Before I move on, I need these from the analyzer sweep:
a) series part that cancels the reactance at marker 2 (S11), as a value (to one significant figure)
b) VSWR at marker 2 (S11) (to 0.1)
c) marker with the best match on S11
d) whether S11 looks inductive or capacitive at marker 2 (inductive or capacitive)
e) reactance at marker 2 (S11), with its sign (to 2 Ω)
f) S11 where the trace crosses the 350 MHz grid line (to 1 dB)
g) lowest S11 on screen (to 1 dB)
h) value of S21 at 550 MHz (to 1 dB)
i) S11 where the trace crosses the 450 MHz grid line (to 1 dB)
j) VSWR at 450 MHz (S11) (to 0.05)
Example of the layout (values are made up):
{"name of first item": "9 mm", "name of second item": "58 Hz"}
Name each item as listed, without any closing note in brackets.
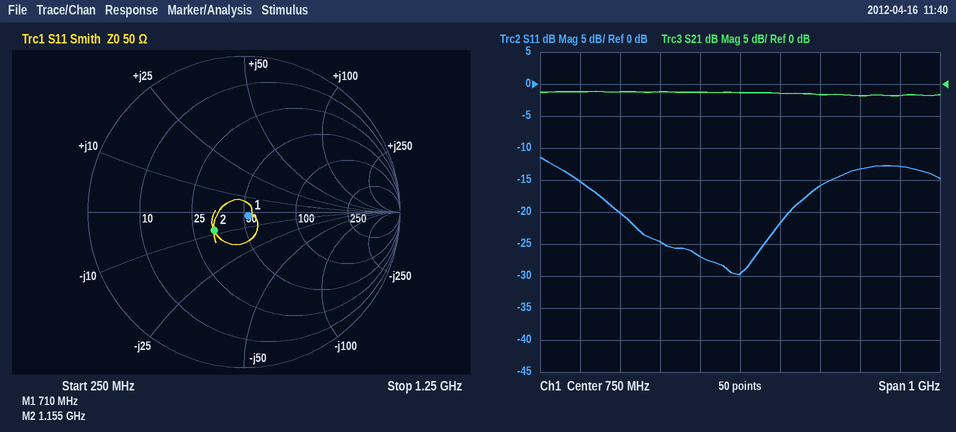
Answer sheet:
{"series part that cancels the reactance at marker 2 (S11), as a value": "1 nH", "VSWR at marker 2 (S11)": "1.6", "marker with the best match on S11": "marker 1", "whether S11 looks inductive or capacitive at marker 2": "capacitive", "reactance at marker 2 (S11), with its sign": "-8 Ω", "S11 where the trace crosses the 350 MHz grid line": "-15 dB", "lowest S11 on screen": "-30 dB", "value of S21 at 550 MHz": "-1 dB", "S11 where the trace crosses the 450 MHz grid line": "-20 dB", "VSWR at 450 MHz (S11)": "1.20"}
